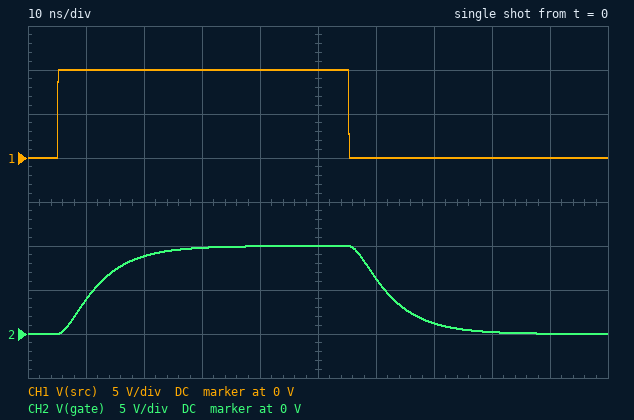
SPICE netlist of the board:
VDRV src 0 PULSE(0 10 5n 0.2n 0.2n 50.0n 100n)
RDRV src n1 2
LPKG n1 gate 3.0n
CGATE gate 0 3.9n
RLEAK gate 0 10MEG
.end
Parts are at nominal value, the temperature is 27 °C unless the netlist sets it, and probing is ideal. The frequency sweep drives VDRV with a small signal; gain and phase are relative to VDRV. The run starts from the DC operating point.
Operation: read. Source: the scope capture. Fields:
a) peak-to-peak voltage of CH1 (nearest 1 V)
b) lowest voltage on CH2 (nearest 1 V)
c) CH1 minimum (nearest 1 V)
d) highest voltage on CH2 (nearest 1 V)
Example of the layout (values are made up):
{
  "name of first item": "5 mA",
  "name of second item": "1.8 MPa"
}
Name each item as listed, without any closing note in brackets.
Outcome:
{
  "peak-to-peak voltage of CH1": "10 V",
  "lowest voltage on CH2": "0 V",
  "CH1 minimum": "0 V",
  "highest voltage on CH2": "10 V"
}
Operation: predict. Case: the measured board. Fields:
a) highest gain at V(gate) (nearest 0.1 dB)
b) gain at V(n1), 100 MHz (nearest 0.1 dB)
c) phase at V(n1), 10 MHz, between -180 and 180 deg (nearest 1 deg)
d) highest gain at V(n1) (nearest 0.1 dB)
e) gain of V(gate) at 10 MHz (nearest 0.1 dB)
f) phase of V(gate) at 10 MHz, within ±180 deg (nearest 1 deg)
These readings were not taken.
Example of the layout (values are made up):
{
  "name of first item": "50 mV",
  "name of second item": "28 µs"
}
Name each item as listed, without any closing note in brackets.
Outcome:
{
  "highest gain at V(gate)": "0 dB",
  "gain at V(n1), 100 MHz": "-4.5 dB",
  "phase at V(n1), 10 MHz, between -180 and 180 deg": "-27 deg",
  "highest gain at V(n1)": "0 dB",
  "gain of V(gate) at 10 MHz": "-0.6 dB",
  "phase of V(gate) at 10 MHz, within ±180 deg": "-27 deg"
}
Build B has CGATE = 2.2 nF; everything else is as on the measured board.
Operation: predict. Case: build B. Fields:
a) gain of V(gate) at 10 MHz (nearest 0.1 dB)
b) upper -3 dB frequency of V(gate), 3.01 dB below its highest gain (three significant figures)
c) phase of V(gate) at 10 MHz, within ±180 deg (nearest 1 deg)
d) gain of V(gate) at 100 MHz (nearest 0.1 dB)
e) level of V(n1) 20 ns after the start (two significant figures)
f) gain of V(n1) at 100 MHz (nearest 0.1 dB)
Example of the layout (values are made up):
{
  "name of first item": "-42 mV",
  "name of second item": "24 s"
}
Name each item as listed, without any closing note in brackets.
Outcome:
{
  "gain of V(gate) at 10 MHz": "-0.1 dB",
  "upper -3 dB frequency of V(gate), 3.01 dB below its highest gain": "49.4 MHz",
  "phase of V(gate) at 10 MHz, within ±180 deg": "-16 deg",
  "gain of V(gate) at 100 MHz": "-10.1 dB",
  "level of V(n1) 20 ns after the start": "10 V",
  "gain of V(n1) at 100 MHz": "-6.0 dB"
}
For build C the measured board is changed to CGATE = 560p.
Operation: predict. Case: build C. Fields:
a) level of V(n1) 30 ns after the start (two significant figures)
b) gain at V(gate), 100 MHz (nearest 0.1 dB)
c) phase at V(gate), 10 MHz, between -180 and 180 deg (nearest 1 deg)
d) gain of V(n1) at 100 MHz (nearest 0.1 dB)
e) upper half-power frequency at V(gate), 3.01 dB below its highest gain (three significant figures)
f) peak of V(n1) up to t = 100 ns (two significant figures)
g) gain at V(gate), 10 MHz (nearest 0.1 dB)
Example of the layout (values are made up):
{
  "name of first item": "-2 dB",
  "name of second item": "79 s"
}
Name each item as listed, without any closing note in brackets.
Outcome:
{
  "level of V(n1) 30 ns after the start": "10 V",
  "gain at V(gate), 100 MHz": "2.2 dB",
  "phase at V(gate), 10 MHz, between -180 and 180 deg": "-4 deg",
  "gain of V(n1) at 100 MHz": "-7.3 dB",
  "upper half-power frequency at V(gate), 3.01 dB below its highest gain": "146 MHz",
  "peak of V(n1) up to t = 100 ns": "11 V",
  "gain at V(gate), 10 MHz": "0 dB"
}
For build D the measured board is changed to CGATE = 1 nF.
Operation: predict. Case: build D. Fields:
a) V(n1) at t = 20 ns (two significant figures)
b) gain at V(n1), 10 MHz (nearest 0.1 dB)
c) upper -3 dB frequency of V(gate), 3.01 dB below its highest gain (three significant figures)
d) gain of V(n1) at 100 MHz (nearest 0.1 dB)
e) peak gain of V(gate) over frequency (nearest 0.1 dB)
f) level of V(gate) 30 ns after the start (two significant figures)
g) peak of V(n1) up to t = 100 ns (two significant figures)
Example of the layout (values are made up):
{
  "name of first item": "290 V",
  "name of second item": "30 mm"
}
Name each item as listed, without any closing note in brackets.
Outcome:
{
  "V(n1) at t = 20 ns": "9.9 V",
  "gain at V(n1), 10 MHz": "-0.1 dB",
  "upper -3 dB frequency of V(gate), 3.01 dB below its highest gain": "104 MHz",
  "gain of V(n1) at 100 MHz": "-16.8 dB",
  "peak gain of V(gate) over frequency": "0.5 dB",
  "level of V(gate) 30 ns after the start": "10 V",
  "peak of V(n1) up to t = 100 ns": "11 V"
}
